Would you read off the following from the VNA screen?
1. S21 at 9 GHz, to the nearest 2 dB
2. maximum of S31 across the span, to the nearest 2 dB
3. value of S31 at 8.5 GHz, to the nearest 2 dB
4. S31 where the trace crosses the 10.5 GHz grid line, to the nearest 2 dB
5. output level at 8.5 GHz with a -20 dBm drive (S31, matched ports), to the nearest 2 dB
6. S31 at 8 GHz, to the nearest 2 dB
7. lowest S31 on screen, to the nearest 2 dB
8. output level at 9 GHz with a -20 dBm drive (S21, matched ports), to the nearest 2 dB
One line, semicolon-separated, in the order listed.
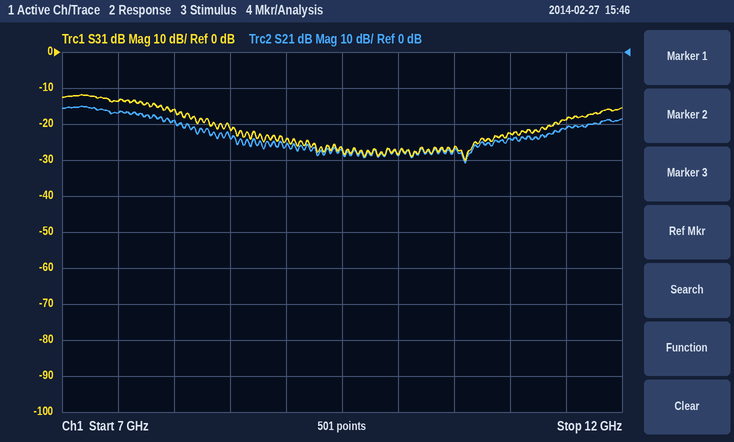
-26 dB; -12 dB; -22 dB; -26 dB; -42 dBm; -16 dB; -30 dB; -46 dBm
